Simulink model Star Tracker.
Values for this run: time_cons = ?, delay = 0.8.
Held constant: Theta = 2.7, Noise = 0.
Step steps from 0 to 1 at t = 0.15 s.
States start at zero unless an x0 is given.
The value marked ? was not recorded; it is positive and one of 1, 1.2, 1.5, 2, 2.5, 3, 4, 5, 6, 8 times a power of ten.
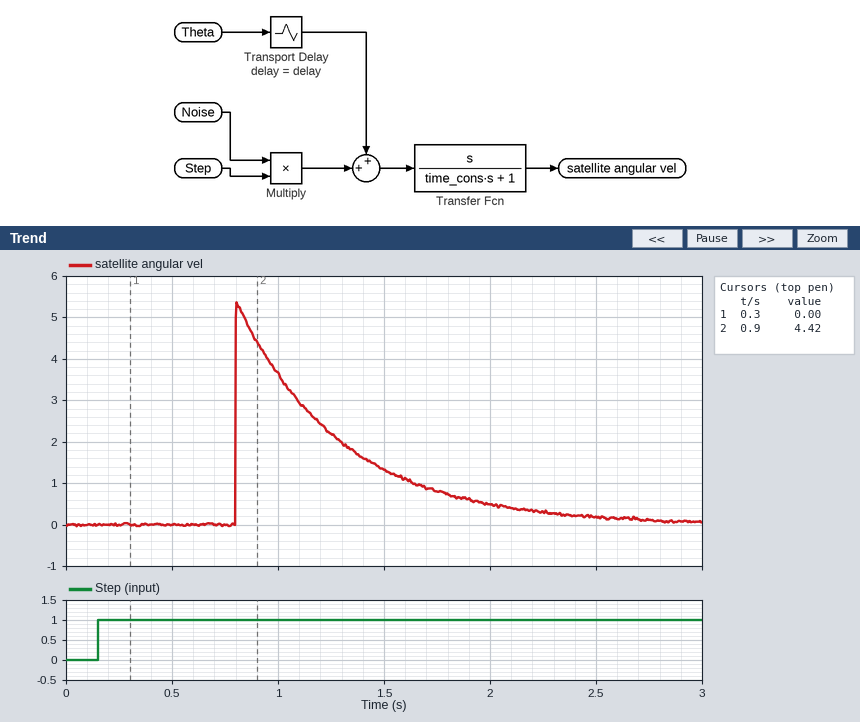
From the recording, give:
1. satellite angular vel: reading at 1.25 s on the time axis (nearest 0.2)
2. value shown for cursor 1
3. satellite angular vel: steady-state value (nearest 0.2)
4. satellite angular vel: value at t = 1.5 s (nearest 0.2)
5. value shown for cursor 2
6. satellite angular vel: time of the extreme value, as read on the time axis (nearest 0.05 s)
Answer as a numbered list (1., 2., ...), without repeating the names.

1. 2.2
2. 0.00
3. 0.0
4. 1.4
5. 4.42
6. 0.80 s
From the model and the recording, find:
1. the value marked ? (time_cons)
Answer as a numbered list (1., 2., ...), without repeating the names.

1. 0.5
